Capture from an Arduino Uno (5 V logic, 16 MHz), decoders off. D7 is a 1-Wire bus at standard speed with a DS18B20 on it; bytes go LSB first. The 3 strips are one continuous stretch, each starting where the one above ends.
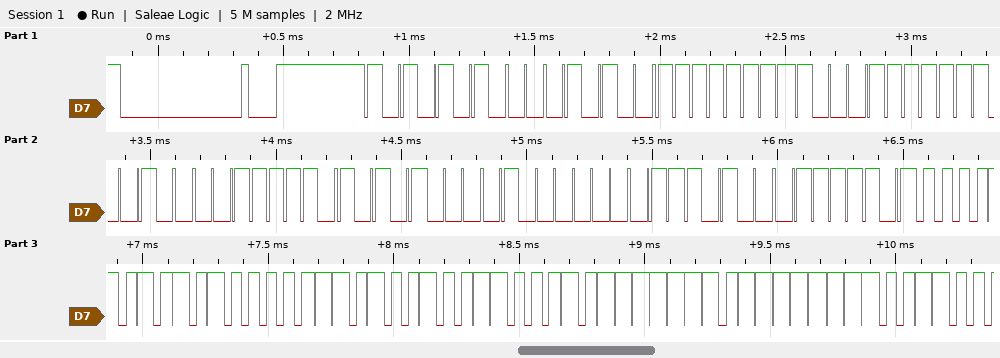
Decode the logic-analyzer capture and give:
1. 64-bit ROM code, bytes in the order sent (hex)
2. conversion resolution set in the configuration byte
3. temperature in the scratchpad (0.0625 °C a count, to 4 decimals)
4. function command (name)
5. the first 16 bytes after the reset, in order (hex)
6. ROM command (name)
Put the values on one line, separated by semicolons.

28 FF F1 27 7C 15 02 2E; 12 bits; 85.0000 °C; Read Scratchpad; 55 28 FF F1 27 7C 15 02 2E BE 50 05 4B 46 7F FF; Match ROM
